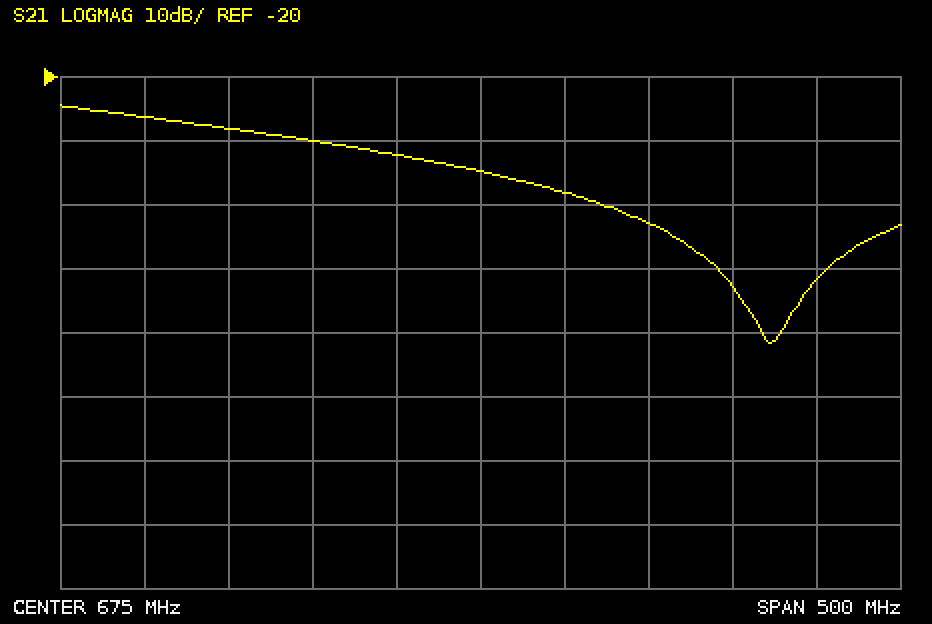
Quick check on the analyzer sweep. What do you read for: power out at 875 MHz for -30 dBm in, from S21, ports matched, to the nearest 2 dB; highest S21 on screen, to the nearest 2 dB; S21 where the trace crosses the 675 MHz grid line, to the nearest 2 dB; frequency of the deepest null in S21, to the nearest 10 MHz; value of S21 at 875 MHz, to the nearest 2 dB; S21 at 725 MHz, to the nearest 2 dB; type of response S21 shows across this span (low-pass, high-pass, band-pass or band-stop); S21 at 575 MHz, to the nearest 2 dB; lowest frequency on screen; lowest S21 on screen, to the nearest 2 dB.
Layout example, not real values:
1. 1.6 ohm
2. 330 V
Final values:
1. -82 dBm
2. -24 dB
3. -34 dB
4. 850 MHz
5. -52 dB
6. -38 dB
7. low-pass
8. -30 dB
9. 425 MHz
10. -62 dB
